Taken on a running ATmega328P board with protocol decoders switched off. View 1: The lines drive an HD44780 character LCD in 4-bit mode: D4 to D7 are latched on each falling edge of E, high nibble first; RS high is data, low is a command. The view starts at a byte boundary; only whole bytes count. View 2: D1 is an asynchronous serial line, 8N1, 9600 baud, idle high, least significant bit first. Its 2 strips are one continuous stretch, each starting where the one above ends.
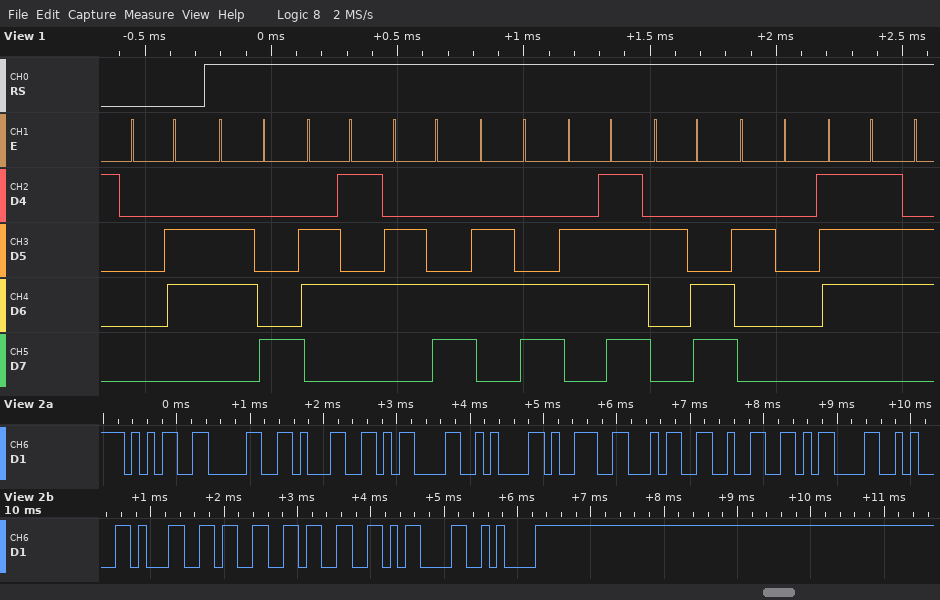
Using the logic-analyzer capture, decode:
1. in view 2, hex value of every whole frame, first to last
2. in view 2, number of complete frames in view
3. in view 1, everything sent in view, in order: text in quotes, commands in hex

0x35 0x30 0x31 0x0D 0x0A 0x39 0x34 0x32 0x0D 0x0A 0x31 0x33 0x33 0x0D 0x0A
15
0x06 "hello, w"
